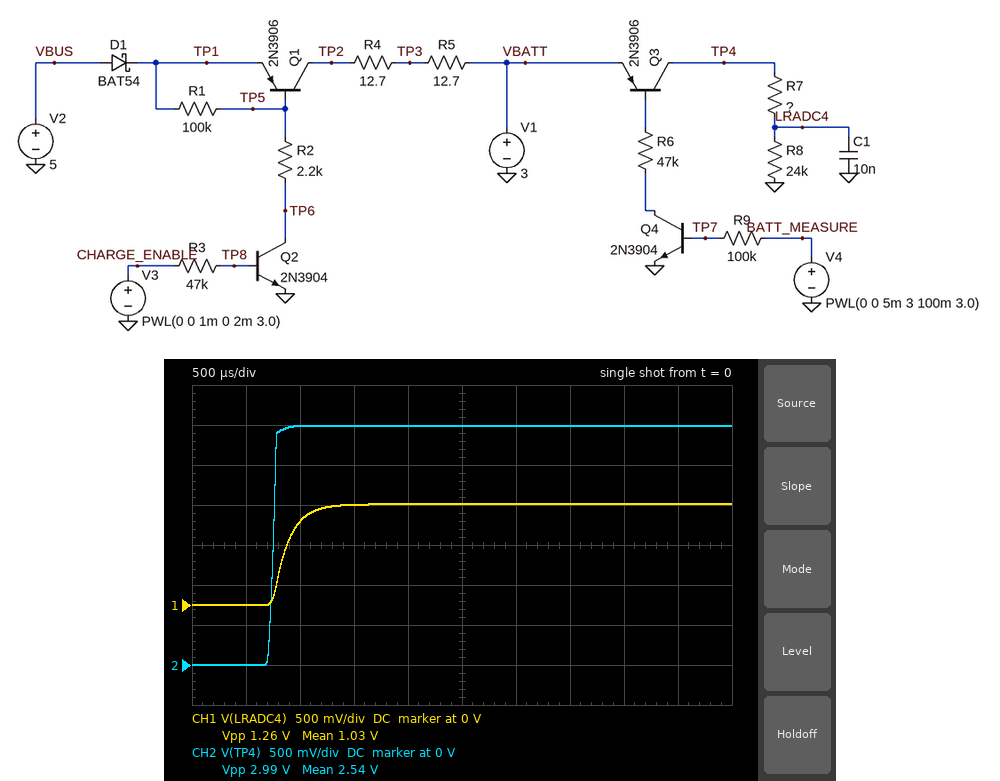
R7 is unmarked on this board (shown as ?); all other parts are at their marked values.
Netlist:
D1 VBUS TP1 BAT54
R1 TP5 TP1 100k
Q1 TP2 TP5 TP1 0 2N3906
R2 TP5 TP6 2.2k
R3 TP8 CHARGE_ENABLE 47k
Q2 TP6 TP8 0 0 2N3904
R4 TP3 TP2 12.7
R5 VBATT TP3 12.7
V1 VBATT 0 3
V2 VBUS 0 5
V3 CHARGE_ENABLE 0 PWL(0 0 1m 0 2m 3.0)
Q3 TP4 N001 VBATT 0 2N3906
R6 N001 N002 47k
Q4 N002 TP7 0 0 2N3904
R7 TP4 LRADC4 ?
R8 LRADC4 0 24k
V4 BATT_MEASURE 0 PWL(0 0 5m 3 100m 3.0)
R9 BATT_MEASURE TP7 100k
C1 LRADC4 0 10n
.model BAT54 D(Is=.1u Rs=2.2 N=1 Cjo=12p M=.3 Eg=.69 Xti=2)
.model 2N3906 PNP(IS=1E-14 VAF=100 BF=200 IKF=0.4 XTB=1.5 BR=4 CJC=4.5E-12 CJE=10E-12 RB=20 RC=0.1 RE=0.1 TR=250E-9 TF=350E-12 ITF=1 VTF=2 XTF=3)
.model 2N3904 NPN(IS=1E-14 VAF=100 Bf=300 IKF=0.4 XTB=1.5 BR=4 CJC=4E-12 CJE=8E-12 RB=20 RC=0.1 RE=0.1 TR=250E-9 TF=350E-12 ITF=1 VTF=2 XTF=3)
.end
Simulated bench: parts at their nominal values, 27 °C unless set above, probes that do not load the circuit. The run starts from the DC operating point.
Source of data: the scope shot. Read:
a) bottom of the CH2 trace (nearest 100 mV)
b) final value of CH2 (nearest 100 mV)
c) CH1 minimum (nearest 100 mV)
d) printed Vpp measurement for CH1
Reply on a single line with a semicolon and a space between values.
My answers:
0 V; 3.0 V; 0 V; 1.26 V
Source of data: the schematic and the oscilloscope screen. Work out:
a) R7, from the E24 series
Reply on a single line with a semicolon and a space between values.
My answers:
33 kΩ
